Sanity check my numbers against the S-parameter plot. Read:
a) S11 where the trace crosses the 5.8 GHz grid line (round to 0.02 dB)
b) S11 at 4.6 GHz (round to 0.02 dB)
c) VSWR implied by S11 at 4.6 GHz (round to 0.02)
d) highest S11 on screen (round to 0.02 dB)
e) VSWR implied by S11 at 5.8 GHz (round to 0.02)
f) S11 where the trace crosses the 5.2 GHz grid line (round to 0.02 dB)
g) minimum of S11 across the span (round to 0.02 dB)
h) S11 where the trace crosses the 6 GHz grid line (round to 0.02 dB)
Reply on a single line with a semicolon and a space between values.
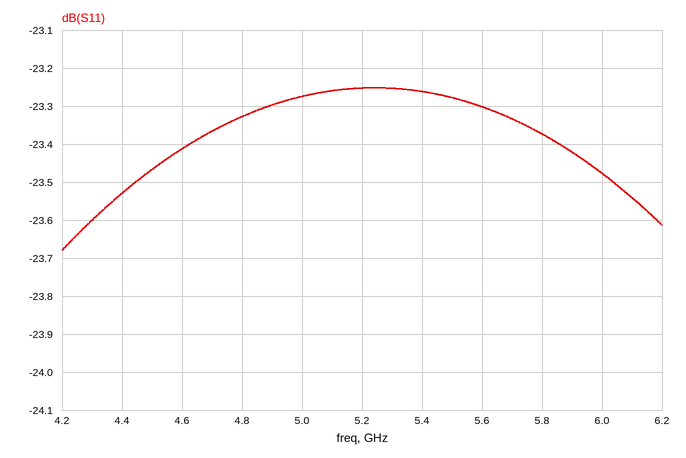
-23.38 dB; -23.42 dB; 1.14; -23.26 dB; 1.14; -23.26 dB; -23.68 dB; -23.48 dB
